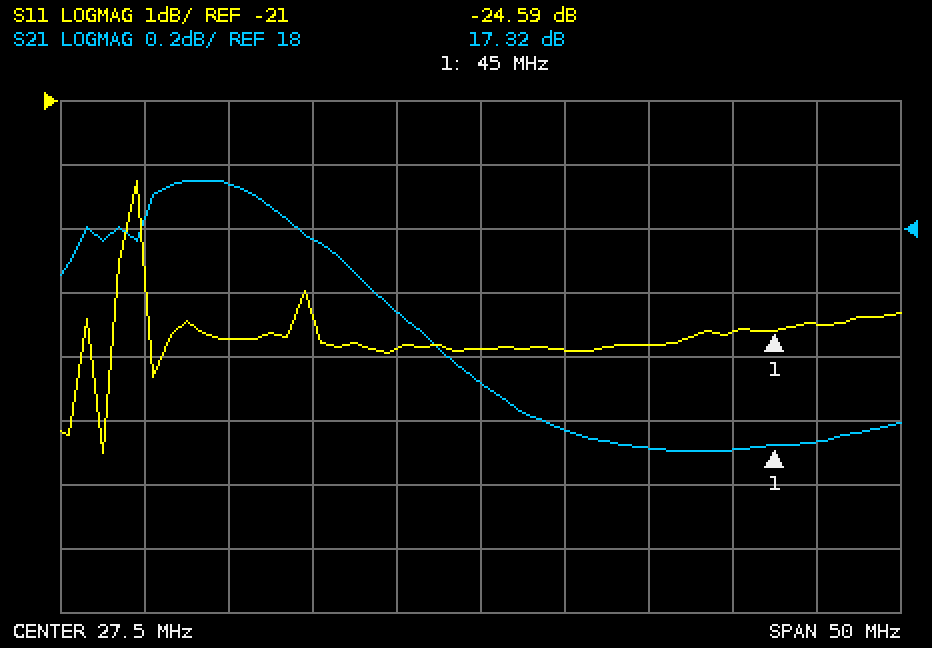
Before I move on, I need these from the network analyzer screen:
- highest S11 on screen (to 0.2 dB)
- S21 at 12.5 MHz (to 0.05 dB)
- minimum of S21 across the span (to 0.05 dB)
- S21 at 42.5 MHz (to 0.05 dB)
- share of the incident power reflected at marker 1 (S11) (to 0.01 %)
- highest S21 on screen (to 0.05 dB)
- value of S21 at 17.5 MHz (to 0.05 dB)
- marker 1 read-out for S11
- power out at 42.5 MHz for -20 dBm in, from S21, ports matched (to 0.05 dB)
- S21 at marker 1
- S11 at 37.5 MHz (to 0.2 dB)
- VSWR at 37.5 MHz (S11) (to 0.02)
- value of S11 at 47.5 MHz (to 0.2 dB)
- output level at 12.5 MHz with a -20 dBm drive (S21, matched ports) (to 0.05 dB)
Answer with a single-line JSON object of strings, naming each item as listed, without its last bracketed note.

{"highest S11 on screen": "-22.2 dB", "S21 at 12.5 MHz": "18.15 dB", "minimum of S21 across the span": "17.30 dB", "S21 at 42.5 MHz": "17.30 dB", "share of the incident power reflected at marker 1 (S11)": "0.35 %", "highest S21 on screen": "18.15 dB", "value of S21 at 17.5 MHz": "17.95 dB", "marker 1 read-out for S11": "-24.59 dB", "power out at 42.5 MHz for -20 dBm in, from S21, ports matched": "-2.70 dBm", "S21 at marker 1": "17.32 dB", "S11 at 37.5 MHz": "-24.8 dB", "VSWR at 37.5 MHz (S11)": "1.12", "value of S11 at 47.5 MHz": "-24.4 dB", "output level at 12.5 MHz with a -20 dBm drive (S21, matched ports)": "-1.85 dBm"}
